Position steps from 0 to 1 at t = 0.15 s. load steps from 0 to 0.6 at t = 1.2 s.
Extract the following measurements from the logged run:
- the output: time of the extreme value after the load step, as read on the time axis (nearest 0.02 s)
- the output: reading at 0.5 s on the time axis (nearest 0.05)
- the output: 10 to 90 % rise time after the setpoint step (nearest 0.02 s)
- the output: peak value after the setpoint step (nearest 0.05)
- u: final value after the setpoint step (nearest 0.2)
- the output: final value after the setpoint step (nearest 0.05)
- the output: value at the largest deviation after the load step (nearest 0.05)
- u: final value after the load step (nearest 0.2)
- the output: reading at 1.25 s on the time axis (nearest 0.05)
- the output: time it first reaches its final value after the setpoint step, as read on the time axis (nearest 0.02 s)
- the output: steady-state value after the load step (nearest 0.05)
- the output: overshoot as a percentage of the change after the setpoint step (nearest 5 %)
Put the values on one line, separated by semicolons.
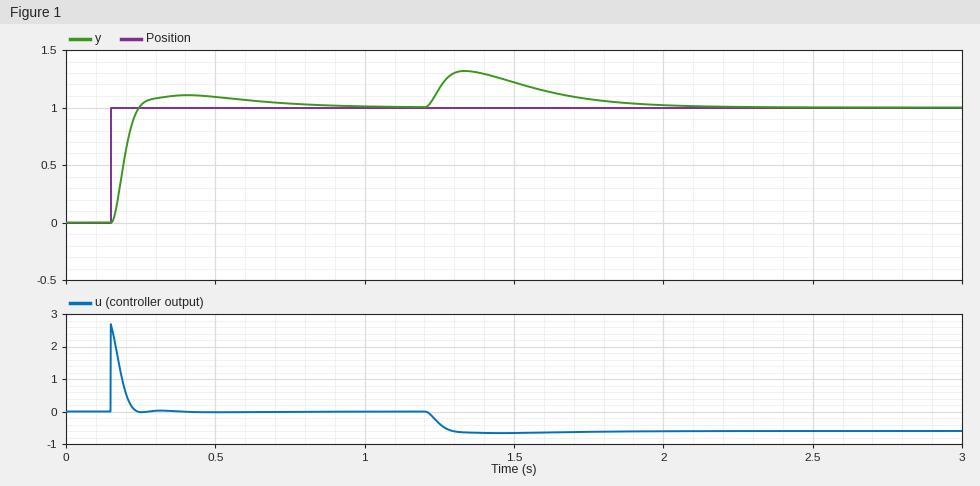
1.34 s; 1.10; 0.06 s; 1.10; 0.0; 1.00; 1.30; -0.6; 1.15; 0.24 s; 1.00; 10 %
